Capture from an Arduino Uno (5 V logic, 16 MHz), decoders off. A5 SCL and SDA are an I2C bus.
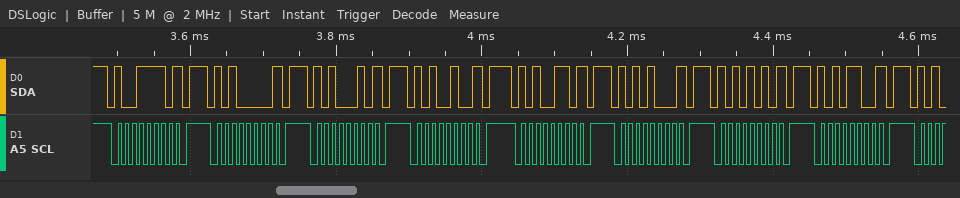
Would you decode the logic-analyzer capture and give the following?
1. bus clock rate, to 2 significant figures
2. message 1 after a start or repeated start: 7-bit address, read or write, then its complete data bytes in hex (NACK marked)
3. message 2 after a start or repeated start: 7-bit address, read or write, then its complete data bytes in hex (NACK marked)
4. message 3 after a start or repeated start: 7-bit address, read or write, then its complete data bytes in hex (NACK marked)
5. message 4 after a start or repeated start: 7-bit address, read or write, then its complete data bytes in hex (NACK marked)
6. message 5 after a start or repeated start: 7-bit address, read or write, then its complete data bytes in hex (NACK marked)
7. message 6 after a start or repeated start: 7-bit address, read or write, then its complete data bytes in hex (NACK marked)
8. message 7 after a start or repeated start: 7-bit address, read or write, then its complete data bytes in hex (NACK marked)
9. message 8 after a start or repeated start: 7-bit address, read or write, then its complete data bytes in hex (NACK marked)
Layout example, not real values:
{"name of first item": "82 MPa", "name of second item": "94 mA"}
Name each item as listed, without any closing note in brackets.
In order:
{"bus clock rate, to 2 significant figures": "100 kHz", "message 1 after a start or repeated start: 7-bit address, read or write, then its complete data bytes in hex": "0x4F write NACK", "message 2 after a start or repeated start: 7-bit address, read or write, then its complete data bytes in hex": "0x50 write NACK", "message 3 after a start or repeated start: 7-bit address, read or write, then its complete data bytes in hex": "0x51 write NACK", "message 4 after a start or repeated start: 7-bit address, read or write, then its complete data bytes in hex": "0x52 write NACK", "message 5 after a start or repeated start: 7-bit address, read or write, then its complete data bytes in hex": "0x53 write NACK", "message 6 after a start or repeated start: 7-bit address, read or write, then its complete data bytes in hex": "0x54 write NACK", "message 7 after a start or repeated start: 7-bit address, read or write, then its complete data bytes in hex": "0x55 write NACK", "message 8 after a start or repeated start: 7-bit address, read or write, then its complete data bytes in hex": "0x56 write NACK"}
